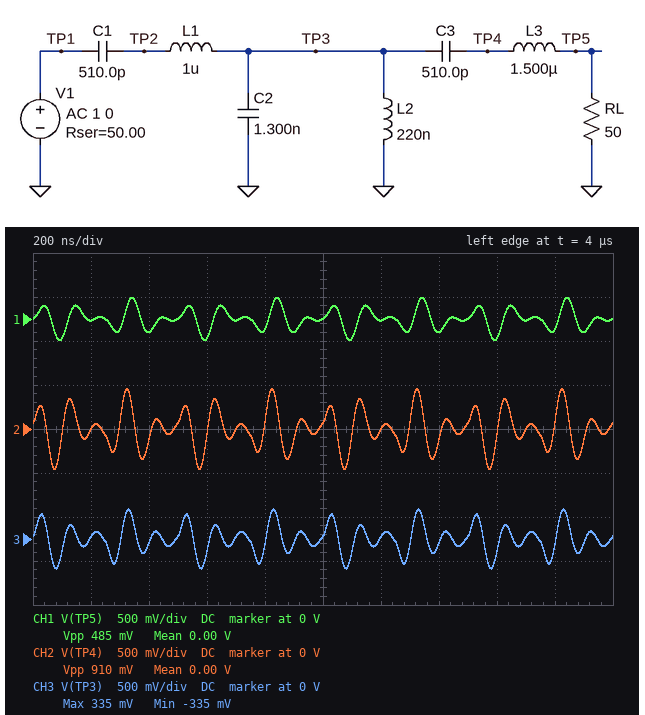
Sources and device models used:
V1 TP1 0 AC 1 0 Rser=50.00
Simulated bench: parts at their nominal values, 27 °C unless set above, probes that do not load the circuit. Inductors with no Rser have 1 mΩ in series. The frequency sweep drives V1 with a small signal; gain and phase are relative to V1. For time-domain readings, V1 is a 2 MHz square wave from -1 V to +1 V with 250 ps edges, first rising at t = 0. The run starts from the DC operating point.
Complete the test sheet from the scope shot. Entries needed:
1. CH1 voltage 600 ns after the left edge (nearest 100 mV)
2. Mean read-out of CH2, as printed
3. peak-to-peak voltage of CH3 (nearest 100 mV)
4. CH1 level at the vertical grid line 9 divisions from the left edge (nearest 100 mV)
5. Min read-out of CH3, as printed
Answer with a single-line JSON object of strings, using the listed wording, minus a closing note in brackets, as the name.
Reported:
{"CH1 voltage 600 ns after the left edge": "-200 mV", "Mean read-out of CH2, as printed": "0.00 V", "peak-to-peak voltage of CH3": "700 mV", "CH1 level at the vertical grid line 9 divisions from the left edge": "-100 mV", "Min read-out of CH3, as printed": "-335 mV"}
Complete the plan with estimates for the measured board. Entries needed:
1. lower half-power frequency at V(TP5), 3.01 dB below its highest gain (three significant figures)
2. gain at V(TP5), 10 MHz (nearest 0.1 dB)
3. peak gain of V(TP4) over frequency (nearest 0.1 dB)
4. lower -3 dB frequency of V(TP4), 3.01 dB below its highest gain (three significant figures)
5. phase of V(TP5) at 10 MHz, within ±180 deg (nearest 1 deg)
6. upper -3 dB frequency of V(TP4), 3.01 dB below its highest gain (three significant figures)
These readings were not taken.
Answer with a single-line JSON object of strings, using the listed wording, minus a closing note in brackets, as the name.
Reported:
{"lower half-power frequency at V(TP5), 3.01 dB below its highest gain": "8.57 MHz", "gain at V(TP5), 10 MHz": "-7.2 dB", "peak gain of V(TP4) over frequency": "0.6 dB", "lower -3 dB frequency of V(TP4), 3.01 dB below its highest gain": "9.25 MHz", "phase of V(TP5) at 10 MHz, within ±180 deg": "-61 deg", "upper -3 dB frequency of V(TP4), 3.01 dB below its highest gain": "11.9 MHz"}
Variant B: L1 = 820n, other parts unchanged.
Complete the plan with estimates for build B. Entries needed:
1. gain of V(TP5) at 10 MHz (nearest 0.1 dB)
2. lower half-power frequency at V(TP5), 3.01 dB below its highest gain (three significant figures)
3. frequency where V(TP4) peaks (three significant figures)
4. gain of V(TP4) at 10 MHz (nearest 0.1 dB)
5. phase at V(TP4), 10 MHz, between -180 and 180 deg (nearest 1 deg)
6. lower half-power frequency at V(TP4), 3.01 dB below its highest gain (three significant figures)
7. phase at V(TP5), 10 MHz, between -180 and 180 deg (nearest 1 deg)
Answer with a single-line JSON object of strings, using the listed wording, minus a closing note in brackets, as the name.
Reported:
{"gain of V(TP5) at 10 MHz": "-7.1 dB", "lower half-power frequency at V(TP5), 3.01 dB below its highest gain": "7.76 MHz", "frequency where V(TP4) peaks": "10.7 MHz", "gain of V(TP4) at 10 MHz": "-0.5 dB", "phase at V(TP4), 10 MHz, between -180 and 180 deg": "5 deg", "lower half-power frequency at V(TP4), 3.01 dB below its highest gain": "8.81 MHz", "phase at V(TP5), 10 MHz, between -180 and 180 deg": "-57 deg"}
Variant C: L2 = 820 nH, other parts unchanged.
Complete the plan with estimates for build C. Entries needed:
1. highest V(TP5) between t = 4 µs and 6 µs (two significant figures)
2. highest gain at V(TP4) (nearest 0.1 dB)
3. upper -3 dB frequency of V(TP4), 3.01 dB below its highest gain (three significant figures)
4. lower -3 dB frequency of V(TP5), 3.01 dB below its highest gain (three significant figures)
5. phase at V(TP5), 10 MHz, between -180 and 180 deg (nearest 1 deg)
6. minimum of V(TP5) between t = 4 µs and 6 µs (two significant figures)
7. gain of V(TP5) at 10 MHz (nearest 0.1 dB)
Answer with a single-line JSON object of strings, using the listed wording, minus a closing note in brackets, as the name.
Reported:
{"highest V(TP5) between t = 4 µs and 6 µs": "250 mV", "highest gain at V(TP4)": "-3.0 dB", "upper -3 dB frequency of V(TP4), 3.01 dB below its highest gain": "9.68 MHz", "lower -3 dB frequency of V(TP5), 3.01 dB below its highest gain": "3.27 MHz", "phase at V(TP5), 10 MHz, between -180 and 180 deg": "-147 deg", "minimum of V(TP5) between t = 4 µs and 6 µs": "-250 mV", "gain of V(TP5) at 10 MHz": "-13.3 dB"}
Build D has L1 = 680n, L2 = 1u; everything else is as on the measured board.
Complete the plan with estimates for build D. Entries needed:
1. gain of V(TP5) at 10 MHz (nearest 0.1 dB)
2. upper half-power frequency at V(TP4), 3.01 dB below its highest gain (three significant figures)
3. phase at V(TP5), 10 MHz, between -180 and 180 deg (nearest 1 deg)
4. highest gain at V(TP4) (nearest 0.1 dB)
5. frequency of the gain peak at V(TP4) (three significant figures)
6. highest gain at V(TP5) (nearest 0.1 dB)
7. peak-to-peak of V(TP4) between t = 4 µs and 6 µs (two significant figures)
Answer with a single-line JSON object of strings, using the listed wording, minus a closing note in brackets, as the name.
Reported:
{"gain of V(TP5) at 10 MHz": "-13.6 dB", "upper half-power frequency at V(TP4), 3.01 dB below its highest gain": "10.2 MHz", "phase at V(TP5), 10 MHz, between -180 and 180 deg": "-127 deg", "highest gain at V(TP4)": "-4.3 dB", "frequency of the gain peak at V(TP4)": "6.98 MHz", "highest gain at V(TP5)": "-6.1 dB", "peak-to-peak of V(TP4) between t = 4 µs and 6 µs": "700 mV"}
